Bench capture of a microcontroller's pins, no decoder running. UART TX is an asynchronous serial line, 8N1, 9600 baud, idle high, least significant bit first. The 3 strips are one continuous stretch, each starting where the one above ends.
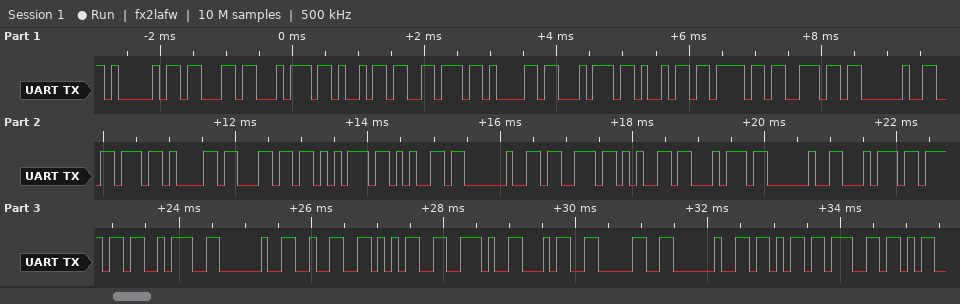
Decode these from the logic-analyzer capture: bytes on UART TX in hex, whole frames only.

41 63 74 69 76 61 74 69 6F 6E 20 76 61 6C 75 65 20 73 65 74 20 74 6F 3A 20 32 35 2E 34 30 20 6B 67
